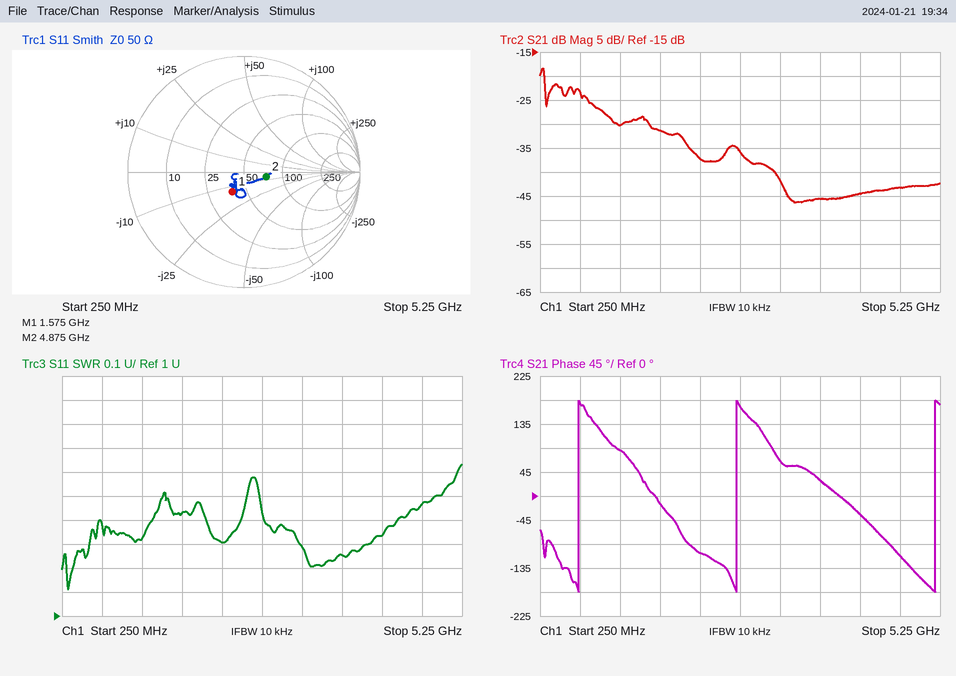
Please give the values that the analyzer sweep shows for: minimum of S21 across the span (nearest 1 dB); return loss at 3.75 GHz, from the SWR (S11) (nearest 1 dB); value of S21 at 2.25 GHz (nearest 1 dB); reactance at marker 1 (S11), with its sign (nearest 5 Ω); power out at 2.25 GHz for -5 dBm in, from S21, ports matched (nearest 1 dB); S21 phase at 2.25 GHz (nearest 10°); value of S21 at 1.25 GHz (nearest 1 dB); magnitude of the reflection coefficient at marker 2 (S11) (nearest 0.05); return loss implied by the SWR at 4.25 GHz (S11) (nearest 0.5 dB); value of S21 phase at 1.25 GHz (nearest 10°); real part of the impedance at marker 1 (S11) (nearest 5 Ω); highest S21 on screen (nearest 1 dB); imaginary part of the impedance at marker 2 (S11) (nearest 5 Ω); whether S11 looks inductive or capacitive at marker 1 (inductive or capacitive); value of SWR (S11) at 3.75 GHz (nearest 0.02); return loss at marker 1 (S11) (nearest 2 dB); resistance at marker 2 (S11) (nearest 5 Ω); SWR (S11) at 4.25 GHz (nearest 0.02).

-46 dB
19 dB
-37 dB
-15 Ω
-42 dBm
-110°
-30 dB
0.20
17.0 dB
90°
40 Ω
-18 dB
-5 Ω
capacitive
1.26
14 dB
75 Ω
1.34
